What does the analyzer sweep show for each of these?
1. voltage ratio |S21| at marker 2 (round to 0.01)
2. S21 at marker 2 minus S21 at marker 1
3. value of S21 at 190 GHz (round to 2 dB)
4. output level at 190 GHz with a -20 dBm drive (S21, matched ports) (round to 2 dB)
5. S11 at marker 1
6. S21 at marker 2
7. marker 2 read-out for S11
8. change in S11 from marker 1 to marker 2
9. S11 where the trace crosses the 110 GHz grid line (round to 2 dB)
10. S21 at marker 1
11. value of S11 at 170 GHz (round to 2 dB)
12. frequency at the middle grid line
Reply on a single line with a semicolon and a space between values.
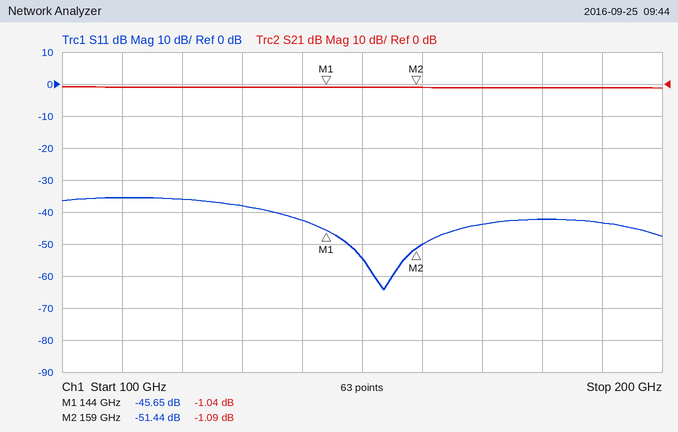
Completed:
0.88; -0.05 dB; -2 dB; -22 dBm; -45.65 dB; -1.09 dB; -51.44 dB; -5.79 dB; -36 dB; -1.04 dB; -44 dB; 150 GHz
